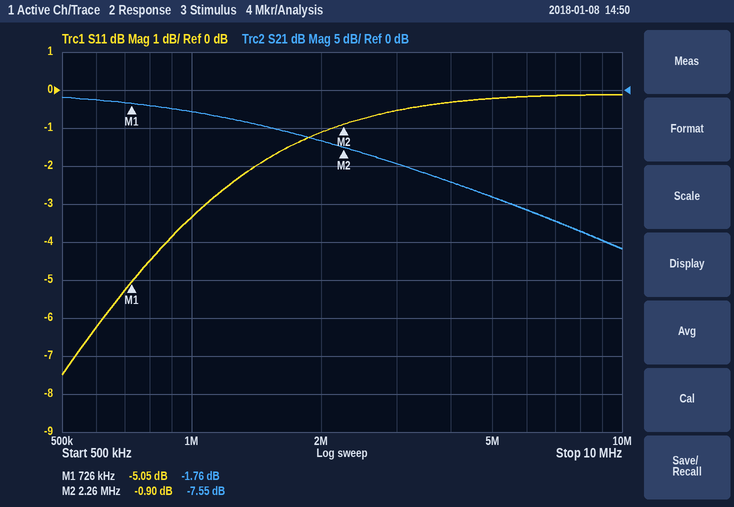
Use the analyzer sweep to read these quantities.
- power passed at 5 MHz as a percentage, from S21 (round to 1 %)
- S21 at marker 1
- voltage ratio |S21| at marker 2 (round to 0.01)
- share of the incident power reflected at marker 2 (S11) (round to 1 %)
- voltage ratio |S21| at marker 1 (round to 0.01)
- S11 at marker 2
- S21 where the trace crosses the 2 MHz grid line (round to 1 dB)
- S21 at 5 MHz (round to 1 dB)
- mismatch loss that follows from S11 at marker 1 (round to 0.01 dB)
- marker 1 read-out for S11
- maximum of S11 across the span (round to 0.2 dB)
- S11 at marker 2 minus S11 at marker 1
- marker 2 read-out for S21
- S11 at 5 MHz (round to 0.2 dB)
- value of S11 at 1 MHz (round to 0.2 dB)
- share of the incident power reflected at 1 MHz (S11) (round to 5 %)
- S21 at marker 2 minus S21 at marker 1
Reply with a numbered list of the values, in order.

1. 4 %
2. -1.76 dB
3. 0.42
4. 81 %
5. 0.82
6. -0.90 dB
7. -7 dB
8. -14 dB
9. 1.63 dB
10. -5.05 dB
11. -0.2 dB
12. 4.15 dB
13. -7.55 dB
14. -0.2 dB
15. -3.4 dB
16. 45 %
17. -5.79 dB
